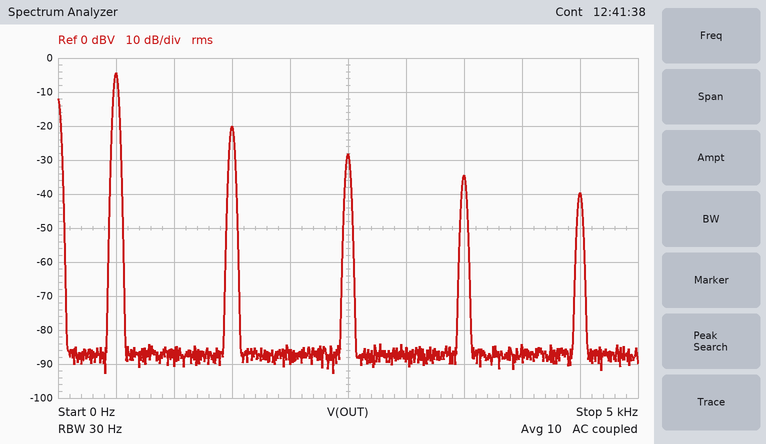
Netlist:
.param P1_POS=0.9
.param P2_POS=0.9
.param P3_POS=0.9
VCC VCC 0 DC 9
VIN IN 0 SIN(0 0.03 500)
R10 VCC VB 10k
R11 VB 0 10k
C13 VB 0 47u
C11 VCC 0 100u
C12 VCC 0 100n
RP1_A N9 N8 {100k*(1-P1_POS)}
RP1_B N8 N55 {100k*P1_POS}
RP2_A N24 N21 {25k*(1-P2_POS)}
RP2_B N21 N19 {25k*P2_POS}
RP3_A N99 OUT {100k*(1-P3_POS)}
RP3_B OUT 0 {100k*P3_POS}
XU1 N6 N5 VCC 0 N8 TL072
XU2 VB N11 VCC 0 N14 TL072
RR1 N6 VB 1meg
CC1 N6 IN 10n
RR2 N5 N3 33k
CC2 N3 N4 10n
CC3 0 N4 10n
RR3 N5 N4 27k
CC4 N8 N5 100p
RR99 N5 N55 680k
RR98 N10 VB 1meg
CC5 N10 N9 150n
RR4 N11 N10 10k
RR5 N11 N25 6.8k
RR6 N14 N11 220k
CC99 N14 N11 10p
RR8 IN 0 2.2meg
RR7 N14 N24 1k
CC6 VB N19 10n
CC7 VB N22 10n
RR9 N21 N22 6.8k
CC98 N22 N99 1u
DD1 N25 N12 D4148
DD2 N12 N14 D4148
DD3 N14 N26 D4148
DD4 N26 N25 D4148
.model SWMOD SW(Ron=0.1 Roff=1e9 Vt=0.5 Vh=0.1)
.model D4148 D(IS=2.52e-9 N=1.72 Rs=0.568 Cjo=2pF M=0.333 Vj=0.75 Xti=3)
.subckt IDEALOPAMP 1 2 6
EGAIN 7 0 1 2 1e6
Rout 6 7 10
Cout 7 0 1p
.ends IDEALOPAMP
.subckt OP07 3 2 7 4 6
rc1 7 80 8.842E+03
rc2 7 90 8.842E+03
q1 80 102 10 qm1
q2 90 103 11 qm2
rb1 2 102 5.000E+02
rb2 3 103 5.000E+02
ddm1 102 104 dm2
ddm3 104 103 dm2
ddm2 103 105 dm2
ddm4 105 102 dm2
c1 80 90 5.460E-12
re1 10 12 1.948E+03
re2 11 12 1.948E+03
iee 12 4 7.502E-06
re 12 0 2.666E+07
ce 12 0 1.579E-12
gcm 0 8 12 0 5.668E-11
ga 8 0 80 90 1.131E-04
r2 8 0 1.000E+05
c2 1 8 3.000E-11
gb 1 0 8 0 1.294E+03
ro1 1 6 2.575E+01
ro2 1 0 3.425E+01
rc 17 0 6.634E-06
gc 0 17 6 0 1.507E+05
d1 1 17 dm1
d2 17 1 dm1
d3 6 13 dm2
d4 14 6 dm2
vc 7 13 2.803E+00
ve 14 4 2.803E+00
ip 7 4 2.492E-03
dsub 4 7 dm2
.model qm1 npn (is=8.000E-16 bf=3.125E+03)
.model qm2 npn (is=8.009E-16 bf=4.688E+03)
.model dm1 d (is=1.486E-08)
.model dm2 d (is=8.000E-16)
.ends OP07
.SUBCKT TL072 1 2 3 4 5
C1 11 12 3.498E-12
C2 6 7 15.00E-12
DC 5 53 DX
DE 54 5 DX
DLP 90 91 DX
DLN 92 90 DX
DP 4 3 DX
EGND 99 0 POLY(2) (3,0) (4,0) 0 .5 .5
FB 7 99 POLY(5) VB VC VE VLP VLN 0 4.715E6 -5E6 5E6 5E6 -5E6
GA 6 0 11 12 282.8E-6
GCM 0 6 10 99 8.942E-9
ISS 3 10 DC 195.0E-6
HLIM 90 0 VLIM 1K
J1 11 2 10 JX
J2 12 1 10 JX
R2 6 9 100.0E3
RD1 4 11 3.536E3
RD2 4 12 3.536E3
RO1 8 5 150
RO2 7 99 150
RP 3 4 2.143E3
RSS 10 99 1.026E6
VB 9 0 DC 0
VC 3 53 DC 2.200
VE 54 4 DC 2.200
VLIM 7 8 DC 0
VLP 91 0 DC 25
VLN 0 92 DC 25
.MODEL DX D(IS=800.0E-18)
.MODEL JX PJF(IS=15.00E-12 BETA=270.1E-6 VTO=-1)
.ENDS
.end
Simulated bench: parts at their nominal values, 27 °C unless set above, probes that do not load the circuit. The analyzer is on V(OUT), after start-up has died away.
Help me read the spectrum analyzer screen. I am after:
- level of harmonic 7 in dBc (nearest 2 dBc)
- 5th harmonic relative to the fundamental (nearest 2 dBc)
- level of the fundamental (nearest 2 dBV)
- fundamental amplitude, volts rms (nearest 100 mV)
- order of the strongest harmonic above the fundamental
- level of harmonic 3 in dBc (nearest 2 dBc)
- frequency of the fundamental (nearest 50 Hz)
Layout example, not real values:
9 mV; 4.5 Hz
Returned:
-30 dBc; -24 dBc; -4 dBV; 600 mV; 3; -16 dBc; 500 Hz
